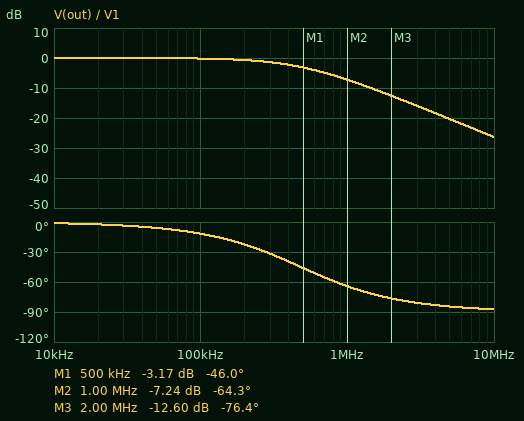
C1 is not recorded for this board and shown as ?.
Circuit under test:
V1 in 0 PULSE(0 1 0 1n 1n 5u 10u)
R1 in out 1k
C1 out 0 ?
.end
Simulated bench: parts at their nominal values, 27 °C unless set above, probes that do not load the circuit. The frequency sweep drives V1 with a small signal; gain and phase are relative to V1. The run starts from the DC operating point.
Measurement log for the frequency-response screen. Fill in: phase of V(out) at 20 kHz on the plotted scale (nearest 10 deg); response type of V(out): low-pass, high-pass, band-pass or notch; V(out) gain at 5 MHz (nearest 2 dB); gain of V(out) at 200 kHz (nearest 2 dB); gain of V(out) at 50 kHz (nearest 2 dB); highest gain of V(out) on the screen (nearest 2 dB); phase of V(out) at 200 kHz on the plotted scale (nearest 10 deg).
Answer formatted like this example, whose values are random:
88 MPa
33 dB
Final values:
0 deg
low-pass
-20 dB
0 dB
0 dB
0 dB
-20 deg
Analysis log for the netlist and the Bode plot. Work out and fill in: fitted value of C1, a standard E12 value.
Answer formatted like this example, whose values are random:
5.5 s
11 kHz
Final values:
330 pF
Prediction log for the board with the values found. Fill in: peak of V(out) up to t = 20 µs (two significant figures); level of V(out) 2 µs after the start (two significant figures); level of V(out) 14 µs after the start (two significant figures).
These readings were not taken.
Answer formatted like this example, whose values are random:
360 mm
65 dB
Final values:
1.0 V
1.0 V
1.0 V
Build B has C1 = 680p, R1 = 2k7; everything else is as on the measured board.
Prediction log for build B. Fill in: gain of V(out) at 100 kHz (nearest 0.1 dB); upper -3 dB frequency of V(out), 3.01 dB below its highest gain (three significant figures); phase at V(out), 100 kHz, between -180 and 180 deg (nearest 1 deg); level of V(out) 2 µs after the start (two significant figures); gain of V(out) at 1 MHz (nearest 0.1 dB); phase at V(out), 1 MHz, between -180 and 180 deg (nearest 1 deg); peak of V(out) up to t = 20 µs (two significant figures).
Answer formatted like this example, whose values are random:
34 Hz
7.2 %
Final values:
-3.7 dB
86.7 kHz
-49 deg
660 mV
-21.3 dB
-85 deg
940 mV
